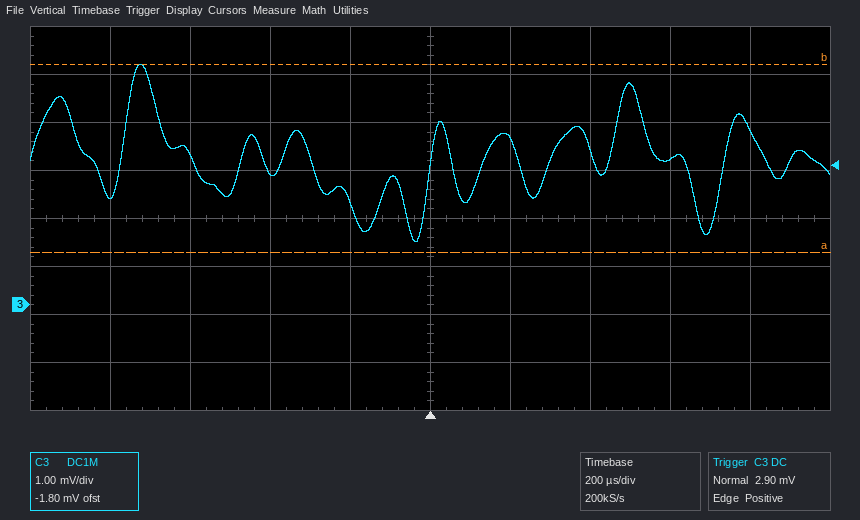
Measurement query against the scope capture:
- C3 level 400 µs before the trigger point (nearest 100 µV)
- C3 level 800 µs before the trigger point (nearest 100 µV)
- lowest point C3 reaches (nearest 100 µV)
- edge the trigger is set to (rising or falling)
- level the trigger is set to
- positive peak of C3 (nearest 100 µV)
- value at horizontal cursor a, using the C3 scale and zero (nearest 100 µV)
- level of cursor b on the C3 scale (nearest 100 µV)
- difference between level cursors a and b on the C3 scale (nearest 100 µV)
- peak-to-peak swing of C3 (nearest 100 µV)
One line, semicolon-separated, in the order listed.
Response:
2.8 mV; 2.3 mV; 1.3 mV; rising; 2.90 mV; 5.0 mV; 1.1 mV; 5.0 mV; 3.9 mV; 3.7 mV
